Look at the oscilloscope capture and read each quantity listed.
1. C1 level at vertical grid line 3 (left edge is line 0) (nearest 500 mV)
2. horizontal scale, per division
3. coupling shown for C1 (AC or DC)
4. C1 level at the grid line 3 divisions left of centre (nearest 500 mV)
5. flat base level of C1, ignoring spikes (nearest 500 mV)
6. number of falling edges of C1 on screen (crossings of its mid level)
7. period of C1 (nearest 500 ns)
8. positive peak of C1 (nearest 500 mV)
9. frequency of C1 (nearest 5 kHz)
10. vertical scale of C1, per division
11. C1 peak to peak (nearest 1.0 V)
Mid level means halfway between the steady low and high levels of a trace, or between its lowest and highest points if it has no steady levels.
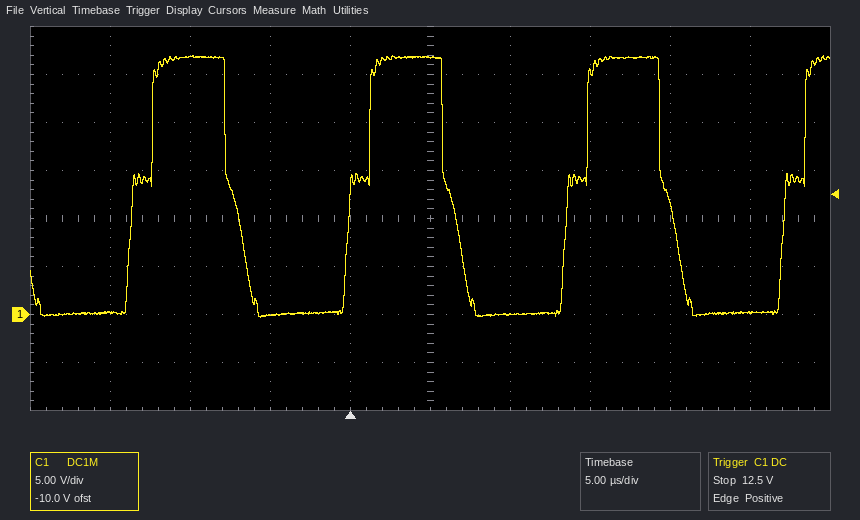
0.0 V
5 µs
DC
27.0 V
0.0 V
3
13.5 µs
27.0 V
75 kHz
5 V
27.0 V
